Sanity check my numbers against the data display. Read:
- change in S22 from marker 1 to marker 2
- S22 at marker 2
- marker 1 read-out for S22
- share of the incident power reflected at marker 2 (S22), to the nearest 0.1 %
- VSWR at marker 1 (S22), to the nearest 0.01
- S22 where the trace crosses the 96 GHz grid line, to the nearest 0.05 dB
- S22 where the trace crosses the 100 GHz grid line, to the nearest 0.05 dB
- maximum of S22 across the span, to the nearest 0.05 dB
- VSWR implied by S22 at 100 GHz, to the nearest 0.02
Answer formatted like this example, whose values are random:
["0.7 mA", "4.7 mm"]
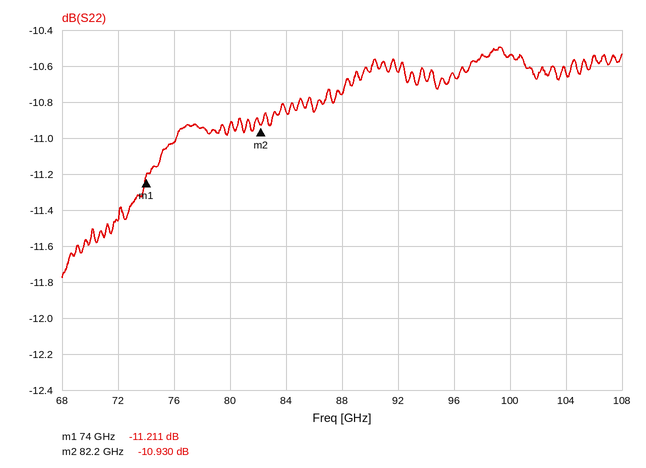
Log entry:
["0.281 dB", "-10.930 dB", "-11.211 dB", "8.1 %", "1.76", "-10.65 dB", "-10.55 dB", "-10.50 dB", "1.84"]
